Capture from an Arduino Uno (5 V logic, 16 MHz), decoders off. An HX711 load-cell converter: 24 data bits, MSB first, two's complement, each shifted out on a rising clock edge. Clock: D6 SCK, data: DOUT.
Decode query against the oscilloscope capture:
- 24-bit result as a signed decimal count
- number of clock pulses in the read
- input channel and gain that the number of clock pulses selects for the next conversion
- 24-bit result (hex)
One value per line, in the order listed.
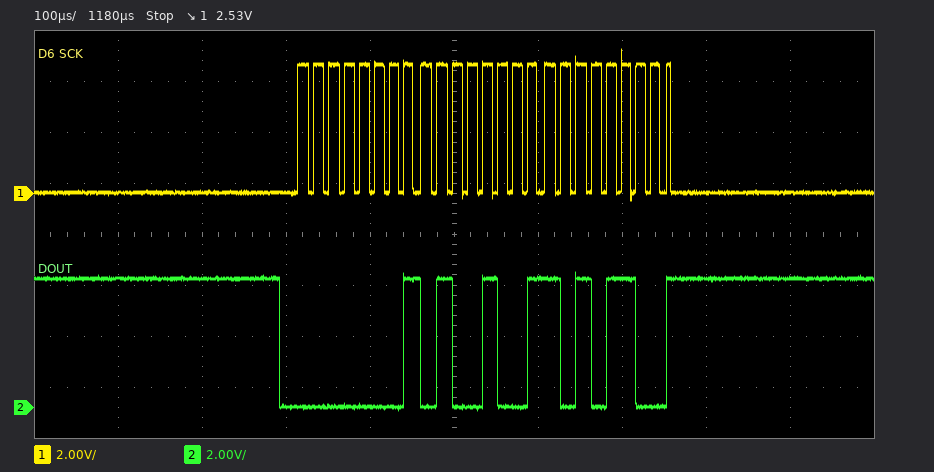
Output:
84396
25
channel A, gain 128
0x0149AC
